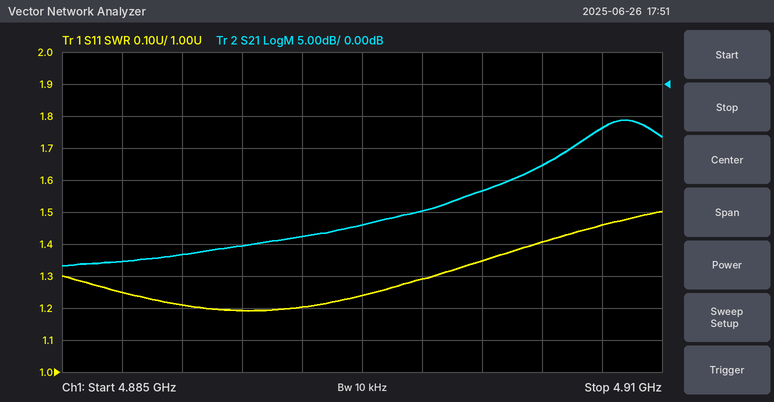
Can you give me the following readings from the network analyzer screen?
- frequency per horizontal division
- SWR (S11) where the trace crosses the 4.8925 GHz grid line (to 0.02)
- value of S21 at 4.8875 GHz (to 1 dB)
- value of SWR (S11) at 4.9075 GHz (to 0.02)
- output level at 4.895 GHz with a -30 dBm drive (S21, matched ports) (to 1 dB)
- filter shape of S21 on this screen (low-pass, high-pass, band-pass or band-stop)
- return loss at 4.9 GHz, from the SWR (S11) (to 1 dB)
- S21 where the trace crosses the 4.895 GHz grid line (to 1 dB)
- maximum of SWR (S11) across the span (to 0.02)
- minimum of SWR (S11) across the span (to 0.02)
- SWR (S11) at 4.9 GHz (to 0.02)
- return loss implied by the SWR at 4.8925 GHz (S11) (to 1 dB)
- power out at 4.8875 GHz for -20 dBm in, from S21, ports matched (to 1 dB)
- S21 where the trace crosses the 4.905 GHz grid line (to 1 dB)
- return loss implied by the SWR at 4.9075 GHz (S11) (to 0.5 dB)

2.5 MHz
1.20
-28 dB
1.46
-54 dBm
high-pass
18 dB
-24 dB
1.50
1.20
1.30
21 dB
-48 dBm
-13 dB
14.5 dB
